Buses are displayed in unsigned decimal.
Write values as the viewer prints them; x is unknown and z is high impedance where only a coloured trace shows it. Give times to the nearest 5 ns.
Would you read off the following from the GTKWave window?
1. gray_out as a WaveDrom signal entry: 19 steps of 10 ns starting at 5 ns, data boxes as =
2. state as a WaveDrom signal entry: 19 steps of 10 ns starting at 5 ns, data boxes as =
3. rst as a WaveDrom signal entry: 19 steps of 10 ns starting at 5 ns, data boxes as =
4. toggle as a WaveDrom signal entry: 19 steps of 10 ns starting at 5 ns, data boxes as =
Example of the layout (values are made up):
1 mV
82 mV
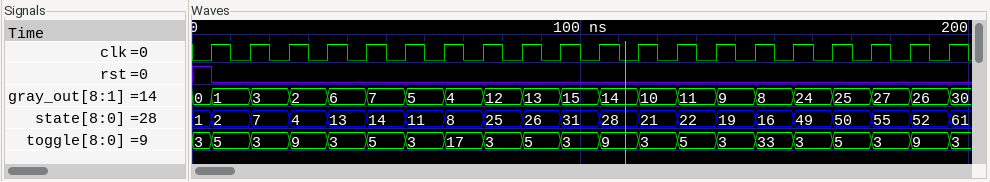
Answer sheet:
{name: 'gray_out', wave: '===================', data: '1 3 2 6 7 5 4 12 13 15 14 10 11 9 8 24 25 27 26'}
{name: 'state', wave: '===================', data: '2 7 4 13 14 11 8 25 26 31 28 21 22 19 16 49 50 55 52'}
{name: 'rst', wave: '0..................'}
{name: 'toggle', wave: '===================', data: '5 3 9 3 5 3 17 3 5 3 9 3 5 3 33 3 5 3 9'}
